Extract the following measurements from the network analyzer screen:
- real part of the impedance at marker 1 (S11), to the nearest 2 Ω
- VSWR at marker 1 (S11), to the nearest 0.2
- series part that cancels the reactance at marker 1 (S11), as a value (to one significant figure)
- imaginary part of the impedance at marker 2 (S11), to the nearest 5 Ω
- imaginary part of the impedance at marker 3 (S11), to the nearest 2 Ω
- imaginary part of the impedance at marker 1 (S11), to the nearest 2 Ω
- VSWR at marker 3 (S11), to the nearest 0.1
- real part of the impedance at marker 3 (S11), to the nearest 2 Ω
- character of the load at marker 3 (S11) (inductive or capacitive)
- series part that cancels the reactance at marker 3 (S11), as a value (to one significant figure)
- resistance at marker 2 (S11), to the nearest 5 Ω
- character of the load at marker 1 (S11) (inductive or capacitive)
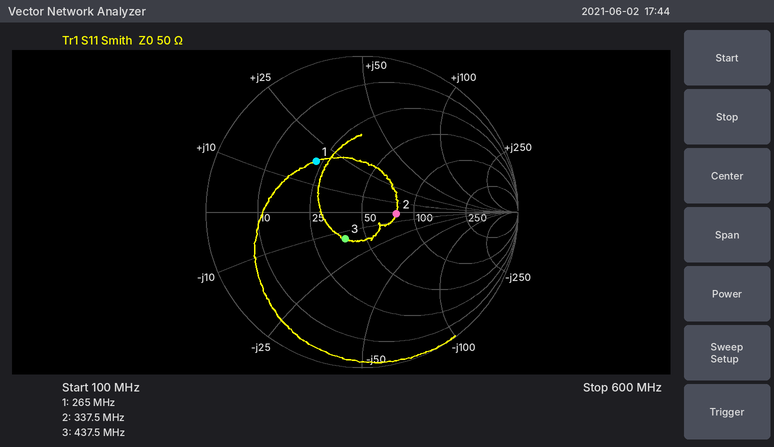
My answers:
22 Ω
2.6
30 pF
0 Ω
-14 Ω
+18 Ω
1.5
38 Ω
capacitive
5 nH
80 Ω
inductive
